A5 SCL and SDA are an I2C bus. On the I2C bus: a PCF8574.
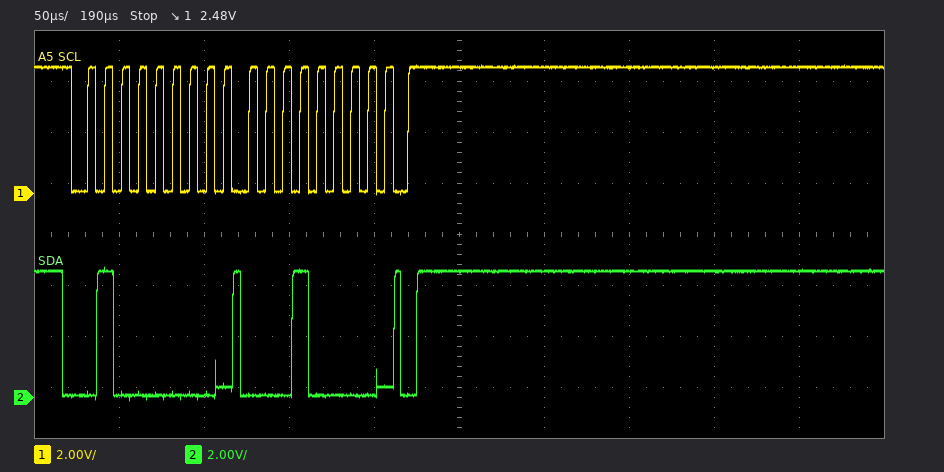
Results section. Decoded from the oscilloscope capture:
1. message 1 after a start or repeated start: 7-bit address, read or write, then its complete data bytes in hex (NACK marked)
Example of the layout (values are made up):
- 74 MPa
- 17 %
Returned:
- 0x20 write: 10
